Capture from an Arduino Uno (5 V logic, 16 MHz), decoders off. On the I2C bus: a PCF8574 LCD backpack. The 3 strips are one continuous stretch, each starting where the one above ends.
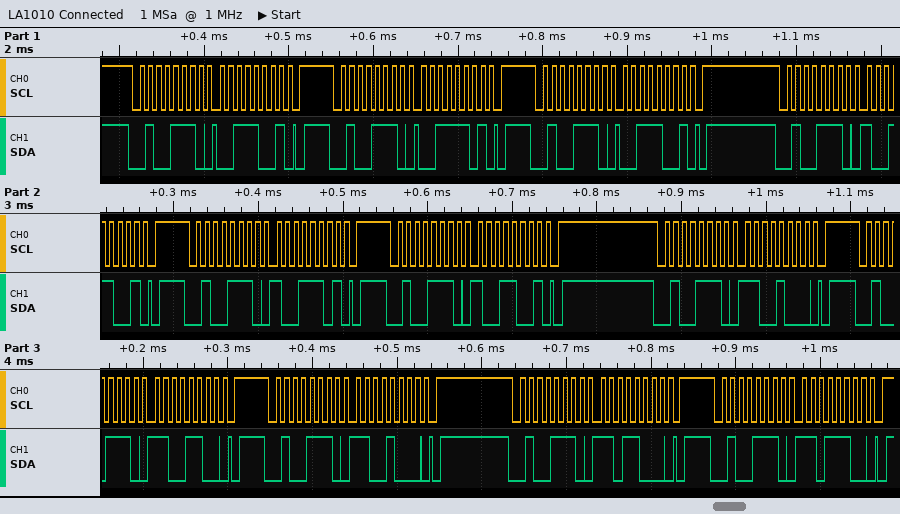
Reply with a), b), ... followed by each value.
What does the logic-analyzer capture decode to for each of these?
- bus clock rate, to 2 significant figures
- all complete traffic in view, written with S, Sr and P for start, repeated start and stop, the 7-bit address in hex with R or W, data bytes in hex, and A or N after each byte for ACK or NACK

a) 100 kHz
b) S 27W A 39 A P S 27W A 3D A P S 27W A 39 A P S 27W A 99 A P S 27W A 9D A P S 27W A 99 A P S 27W A C8 A P S 27W A CC A P S 27W A C8 A P S 27W A D8 A P S 27W A DC A P
